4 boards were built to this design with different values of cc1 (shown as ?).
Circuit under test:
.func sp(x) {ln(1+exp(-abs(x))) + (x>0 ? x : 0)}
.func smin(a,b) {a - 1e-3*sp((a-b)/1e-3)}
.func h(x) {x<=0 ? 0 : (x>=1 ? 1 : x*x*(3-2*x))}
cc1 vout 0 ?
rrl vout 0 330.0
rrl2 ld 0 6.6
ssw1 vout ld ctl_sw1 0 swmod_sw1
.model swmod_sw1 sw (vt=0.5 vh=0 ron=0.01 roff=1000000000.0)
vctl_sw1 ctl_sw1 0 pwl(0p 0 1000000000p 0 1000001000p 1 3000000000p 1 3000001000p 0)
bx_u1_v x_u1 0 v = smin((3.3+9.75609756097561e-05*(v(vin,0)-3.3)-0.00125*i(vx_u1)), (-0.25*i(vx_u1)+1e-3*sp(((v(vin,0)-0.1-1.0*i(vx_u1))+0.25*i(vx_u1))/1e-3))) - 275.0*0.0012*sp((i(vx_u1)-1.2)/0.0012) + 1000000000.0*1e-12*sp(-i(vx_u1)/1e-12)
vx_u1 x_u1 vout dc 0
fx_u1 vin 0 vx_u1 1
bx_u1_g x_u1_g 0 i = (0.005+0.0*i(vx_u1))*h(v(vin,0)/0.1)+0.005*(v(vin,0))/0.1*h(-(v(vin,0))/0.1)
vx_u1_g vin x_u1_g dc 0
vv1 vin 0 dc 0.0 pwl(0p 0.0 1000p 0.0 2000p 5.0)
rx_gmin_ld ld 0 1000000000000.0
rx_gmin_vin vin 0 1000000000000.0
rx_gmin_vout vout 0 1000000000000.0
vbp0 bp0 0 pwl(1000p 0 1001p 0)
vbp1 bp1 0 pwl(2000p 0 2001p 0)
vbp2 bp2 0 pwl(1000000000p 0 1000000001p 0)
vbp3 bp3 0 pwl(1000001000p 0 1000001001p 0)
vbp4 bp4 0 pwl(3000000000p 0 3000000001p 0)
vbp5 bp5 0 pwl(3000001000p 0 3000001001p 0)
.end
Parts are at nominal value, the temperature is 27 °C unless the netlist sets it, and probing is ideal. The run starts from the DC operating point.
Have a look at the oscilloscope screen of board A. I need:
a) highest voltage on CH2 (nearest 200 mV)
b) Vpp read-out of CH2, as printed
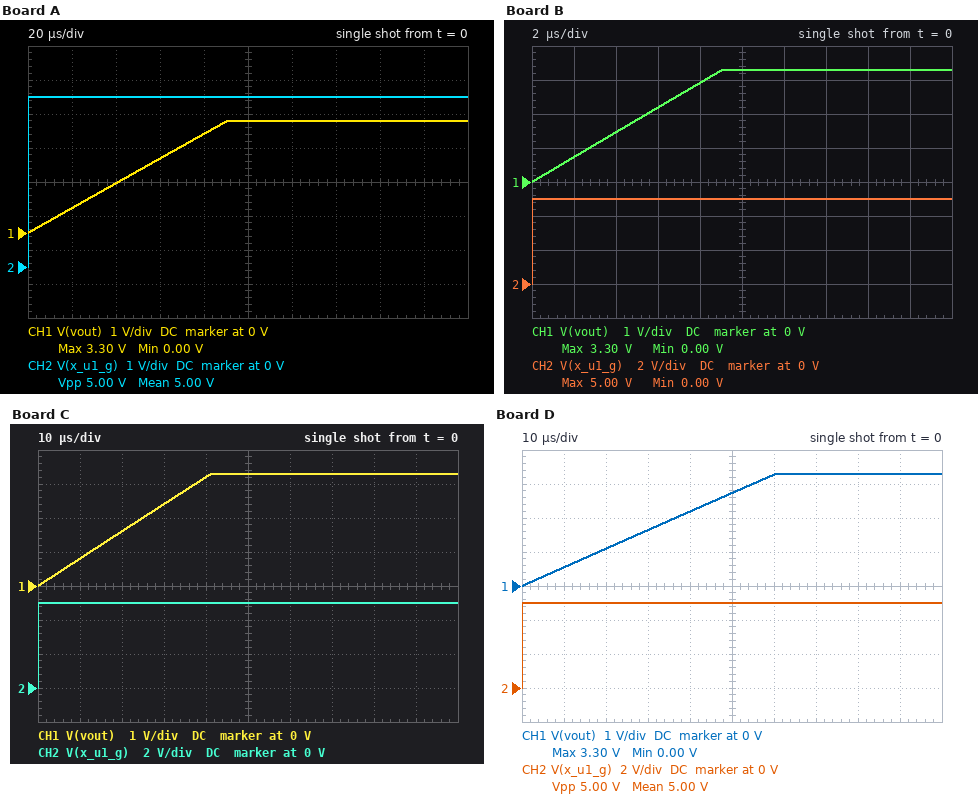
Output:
5.0 V
5.00 V
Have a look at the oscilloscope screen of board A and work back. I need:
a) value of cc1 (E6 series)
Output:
33 µF
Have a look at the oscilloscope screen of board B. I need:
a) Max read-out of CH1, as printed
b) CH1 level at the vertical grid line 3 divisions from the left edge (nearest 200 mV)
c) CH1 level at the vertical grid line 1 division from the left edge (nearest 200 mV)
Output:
3.30 V
2.2 V
800 mV
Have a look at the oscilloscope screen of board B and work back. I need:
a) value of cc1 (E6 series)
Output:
3.3 µF
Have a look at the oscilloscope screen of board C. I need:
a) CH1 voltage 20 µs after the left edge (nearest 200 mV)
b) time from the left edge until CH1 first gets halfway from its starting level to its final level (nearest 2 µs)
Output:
1.6 V
20 µs
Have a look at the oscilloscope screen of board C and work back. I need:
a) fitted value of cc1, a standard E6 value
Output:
15 µF
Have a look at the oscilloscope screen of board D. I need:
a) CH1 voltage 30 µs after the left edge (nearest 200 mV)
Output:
1.6 V
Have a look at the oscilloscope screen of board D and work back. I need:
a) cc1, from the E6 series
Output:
22 µF
